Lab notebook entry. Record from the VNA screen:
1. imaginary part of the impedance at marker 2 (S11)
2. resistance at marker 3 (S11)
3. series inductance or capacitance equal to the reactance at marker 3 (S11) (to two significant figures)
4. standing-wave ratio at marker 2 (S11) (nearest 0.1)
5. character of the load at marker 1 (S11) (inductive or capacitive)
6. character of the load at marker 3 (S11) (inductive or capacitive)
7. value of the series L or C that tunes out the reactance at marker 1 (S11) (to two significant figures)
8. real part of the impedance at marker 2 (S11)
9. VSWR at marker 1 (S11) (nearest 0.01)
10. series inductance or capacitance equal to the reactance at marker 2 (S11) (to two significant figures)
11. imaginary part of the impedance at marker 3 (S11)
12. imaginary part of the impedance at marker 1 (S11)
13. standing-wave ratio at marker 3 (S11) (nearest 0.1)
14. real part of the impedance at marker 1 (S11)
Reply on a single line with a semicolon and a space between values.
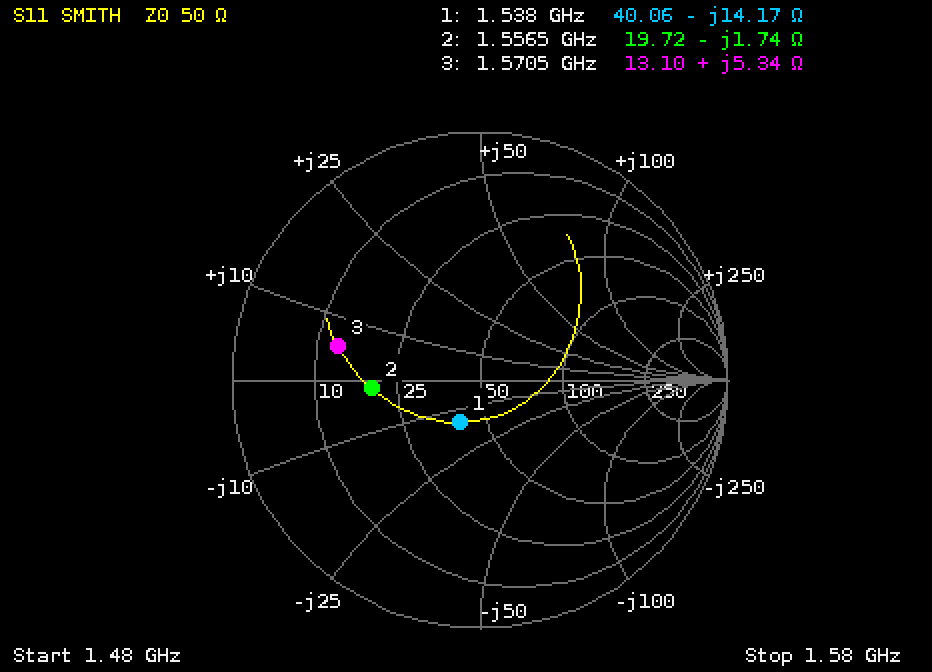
-1.74 Ω; 13.10 Ω; 540 pH; 2.5; capacitive; inductive; 1.5 nH; 19.72 Ω; 1.47; 59 pF; +5.34 Ω; -14.17 Ω; 3.9; 40.06 Ω
